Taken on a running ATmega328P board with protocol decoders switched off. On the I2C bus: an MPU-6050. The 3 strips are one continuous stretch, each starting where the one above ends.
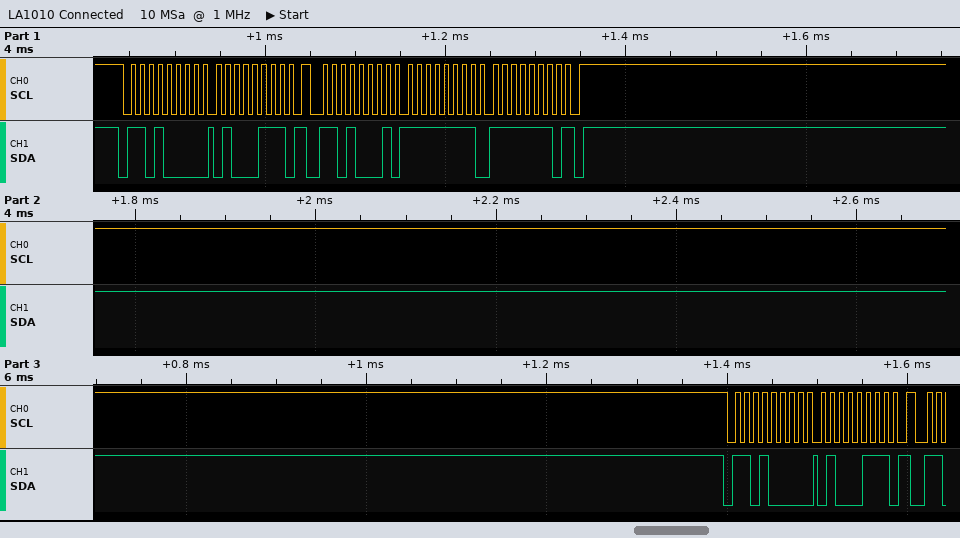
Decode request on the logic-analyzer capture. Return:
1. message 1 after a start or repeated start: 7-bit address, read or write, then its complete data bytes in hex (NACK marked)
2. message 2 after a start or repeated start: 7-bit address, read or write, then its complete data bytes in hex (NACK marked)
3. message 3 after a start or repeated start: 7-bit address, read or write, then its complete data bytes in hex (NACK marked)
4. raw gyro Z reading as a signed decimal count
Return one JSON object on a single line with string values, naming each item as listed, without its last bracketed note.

{"message 1 after a start or repeated start: 7-bit address, read or write, then its complete data bytes in hex": "0x68 write: 47", "message 2 after a start or repeated start: 7-bit address, read or write, then its complete data bytes in hex": "0x68 read: FF FE NACK", "message 3 after a start or repeated start: 7-bit address, read or write, then its complete data bytes in hex": "0x68 write: 47", "raw gyro Z reading as a signed decimal count": "-2"}
